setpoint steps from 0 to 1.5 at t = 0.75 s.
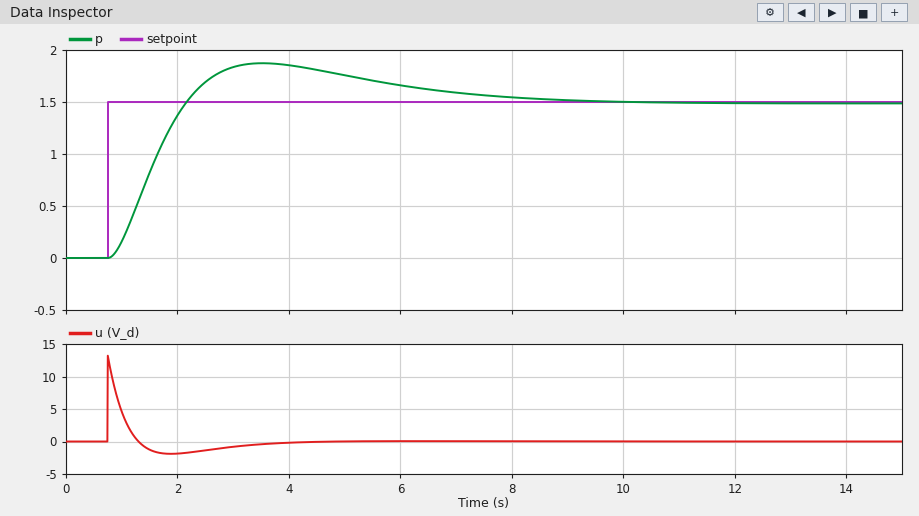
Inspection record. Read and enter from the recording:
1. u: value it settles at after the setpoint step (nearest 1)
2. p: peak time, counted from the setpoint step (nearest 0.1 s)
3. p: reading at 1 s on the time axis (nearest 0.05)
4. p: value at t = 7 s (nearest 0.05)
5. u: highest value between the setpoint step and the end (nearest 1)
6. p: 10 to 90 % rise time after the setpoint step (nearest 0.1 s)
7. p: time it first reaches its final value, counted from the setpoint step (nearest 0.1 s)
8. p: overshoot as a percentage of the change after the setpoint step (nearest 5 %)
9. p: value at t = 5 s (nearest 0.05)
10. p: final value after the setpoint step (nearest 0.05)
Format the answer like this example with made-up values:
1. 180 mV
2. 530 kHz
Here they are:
1. 0
2. 2.8 s
3. 0.15
4. 1.60
5. 13
6. 1.0 s
7. 1.4 s
8. 25 %
9. 1.75
10. 1.50
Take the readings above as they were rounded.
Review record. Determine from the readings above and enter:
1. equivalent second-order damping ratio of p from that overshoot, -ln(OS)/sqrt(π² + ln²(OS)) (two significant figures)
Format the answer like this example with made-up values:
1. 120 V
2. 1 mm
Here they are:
1. 0.40
